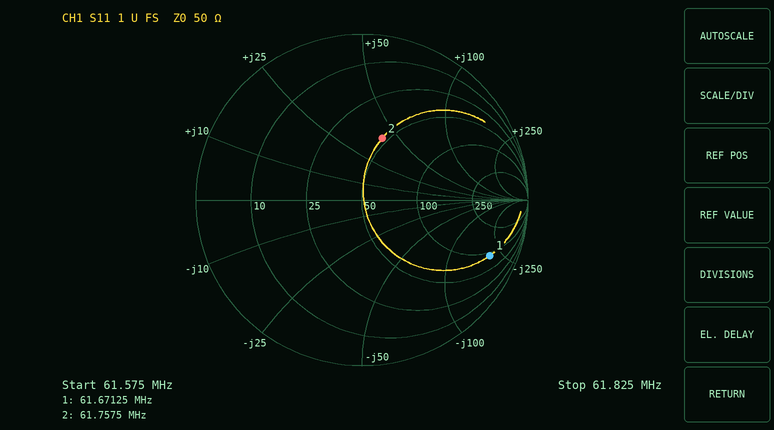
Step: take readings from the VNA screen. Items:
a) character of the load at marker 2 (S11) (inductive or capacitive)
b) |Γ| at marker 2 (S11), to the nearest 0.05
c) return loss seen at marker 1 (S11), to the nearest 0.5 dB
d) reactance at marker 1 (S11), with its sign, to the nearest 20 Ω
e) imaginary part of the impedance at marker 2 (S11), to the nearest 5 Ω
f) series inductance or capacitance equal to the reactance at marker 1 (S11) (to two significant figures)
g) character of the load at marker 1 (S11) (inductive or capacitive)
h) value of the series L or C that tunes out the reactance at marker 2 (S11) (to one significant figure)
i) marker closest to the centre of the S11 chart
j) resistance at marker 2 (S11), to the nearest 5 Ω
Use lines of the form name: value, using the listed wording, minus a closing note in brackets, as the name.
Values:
character of the load at marker 2 (S11): inductive
|Γ| at marker 2 (S11), to the nearest 0.05: 0.40
return loss seen at marker 1 (S11), to the nearest 0.5 dB: 1.5 dB
reactance at marker 1 (S11), with its sign, to the nearest 20 Ω: -200 Ω
imaginary part of the impedance at marker 2 (S11), to the nearest 5 Ω: +40 Ω
series inductance or capacitance equal to the reactance at marker 1 (S11): 13 pF
character of the load at marker 1 (S11): capacitive
value of the series L or C that tunes out the reactance at marker 2 (S11): 60 pF
marker closest to the centre of the S11 chart: marker 2
resistance at marker 2 (S11), to the nearest 5 Ω: 45 Ω
